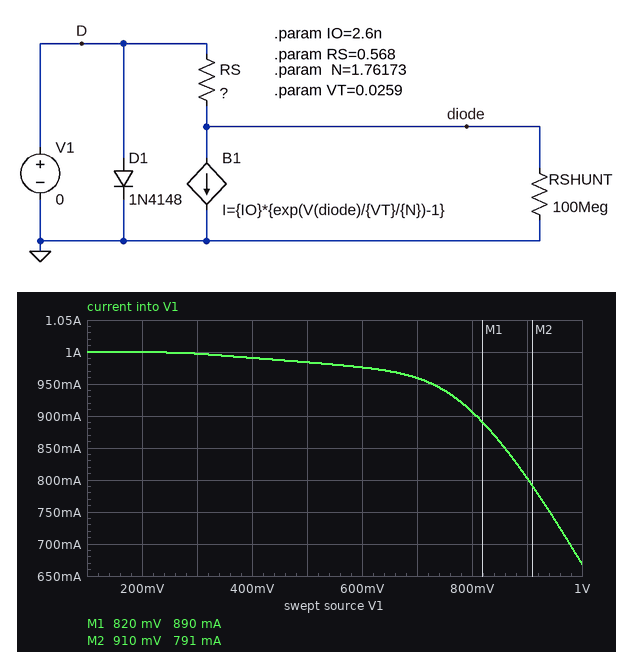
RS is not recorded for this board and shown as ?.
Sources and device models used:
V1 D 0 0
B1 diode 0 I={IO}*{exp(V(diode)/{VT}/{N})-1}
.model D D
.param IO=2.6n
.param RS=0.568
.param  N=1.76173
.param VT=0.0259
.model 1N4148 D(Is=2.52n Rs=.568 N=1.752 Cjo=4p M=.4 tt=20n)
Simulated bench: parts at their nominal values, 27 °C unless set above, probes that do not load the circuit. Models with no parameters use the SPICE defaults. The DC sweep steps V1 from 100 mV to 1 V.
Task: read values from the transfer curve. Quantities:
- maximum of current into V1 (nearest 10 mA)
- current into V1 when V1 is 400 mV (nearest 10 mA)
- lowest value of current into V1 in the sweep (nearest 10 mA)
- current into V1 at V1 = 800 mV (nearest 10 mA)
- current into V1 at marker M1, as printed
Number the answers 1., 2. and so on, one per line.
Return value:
1. 1.00 A
2. 990 mA
3. 670 mA
4. 910 mA
5. 890 mA
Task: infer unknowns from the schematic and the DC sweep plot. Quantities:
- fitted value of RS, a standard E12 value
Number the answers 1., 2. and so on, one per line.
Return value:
1. 0.33 Ω
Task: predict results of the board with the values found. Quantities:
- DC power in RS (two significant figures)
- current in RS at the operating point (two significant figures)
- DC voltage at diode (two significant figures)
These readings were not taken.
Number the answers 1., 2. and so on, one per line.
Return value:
1. 330 mW
2. 1.0 A
3. 330 mV
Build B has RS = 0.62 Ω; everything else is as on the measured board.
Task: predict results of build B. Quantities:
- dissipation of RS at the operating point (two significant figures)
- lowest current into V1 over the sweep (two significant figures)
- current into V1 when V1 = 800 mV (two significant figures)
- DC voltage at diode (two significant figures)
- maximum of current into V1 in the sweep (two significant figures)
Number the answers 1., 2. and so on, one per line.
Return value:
1. 620 mW
2. 650 mA
3. 890 mA
4. 620 mV
5. 990 mA
